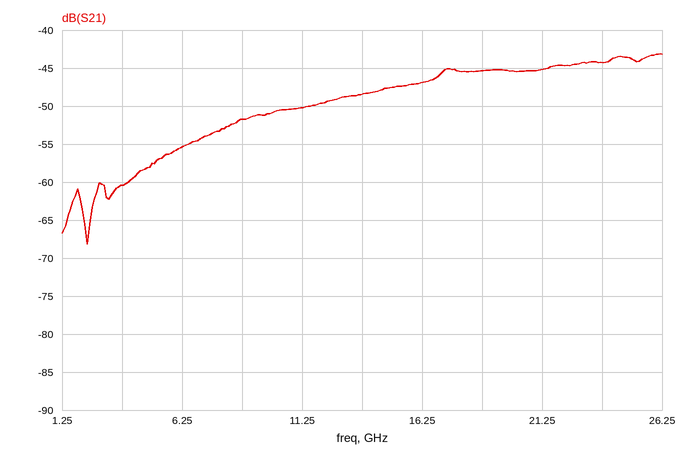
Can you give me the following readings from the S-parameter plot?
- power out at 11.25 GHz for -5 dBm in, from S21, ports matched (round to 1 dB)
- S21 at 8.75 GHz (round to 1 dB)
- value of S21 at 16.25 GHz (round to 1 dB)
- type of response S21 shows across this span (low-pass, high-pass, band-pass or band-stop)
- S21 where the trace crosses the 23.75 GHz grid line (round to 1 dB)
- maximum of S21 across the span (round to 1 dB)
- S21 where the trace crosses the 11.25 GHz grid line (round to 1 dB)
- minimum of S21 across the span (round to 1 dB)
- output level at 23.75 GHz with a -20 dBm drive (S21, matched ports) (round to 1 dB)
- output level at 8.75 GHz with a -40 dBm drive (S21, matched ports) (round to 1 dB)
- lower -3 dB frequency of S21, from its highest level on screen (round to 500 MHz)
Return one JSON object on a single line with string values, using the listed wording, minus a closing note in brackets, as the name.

{"power out at 11.25 GHz for -5 dBm in, from S21, ports matched": "-55 dBm", "S21 at 8.75 GHz": "-52 dB", "value of S21 at 16.25 GHz": "-47 dB", "type of response S21 shows across this span": "high-pass", "S21 where the trace crosses the 23.75 GHz grid line": "-44 dB", "maximum of S21 across the span": "-43 dB", "S21 where the trace crosses the 11.25 GHz grid line": "-50 dB", "minimum of S21 across the span": "-68 dB", "output level at 23.75 GHz with a -20 dBm drive (S21, matched ports)": "-64 dBm", "output level at 8.75 GHz with a -40 dBm drive (S21, matched ports)": "-92 dBm", "lower -3 dB frequency of S21, from its highest level on screen": "17.0 GHz"}
